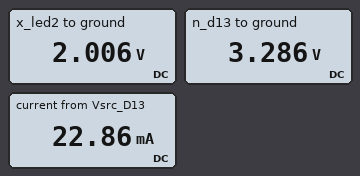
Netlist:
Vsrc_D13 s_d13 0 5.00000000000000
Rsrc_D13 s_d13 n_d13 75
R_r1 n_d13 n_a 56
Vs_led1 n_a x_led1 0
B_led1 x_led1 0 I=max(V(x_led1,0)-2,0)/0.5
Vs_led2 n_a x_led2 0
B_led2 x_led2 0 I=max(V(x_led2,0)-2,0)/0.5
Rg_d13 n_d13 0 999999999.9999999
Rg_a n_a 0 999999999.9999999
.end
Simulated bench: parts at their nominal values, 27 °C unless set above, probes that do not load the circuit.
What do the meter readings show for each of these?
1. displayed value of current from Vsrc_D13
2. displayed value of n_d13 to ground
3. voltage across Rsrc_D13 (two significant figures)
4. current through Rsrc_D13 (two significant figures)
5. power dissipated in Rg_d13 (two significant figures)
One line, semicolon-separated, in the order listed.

22.86 mA; 3.286 V; 1.7 V; 23 mA; 11 nW
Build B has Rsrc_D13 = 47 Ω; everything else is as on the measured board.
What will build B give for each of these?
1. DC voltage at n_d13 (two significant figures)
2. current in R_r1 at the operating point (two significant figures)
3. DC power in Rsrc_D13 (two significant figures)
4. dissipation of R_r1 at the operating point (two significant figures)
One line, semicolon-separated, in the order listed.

3.6 V; 29 mA; 40 mW; 47 mW
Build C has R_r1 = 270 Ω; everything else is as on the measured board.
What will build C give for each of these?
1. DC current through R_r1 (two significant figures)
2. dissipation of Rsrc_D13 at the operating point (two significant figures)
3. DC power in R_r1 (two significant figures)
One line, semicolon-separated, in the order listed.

8.7 mA; 5.7 mW; 20 mW
